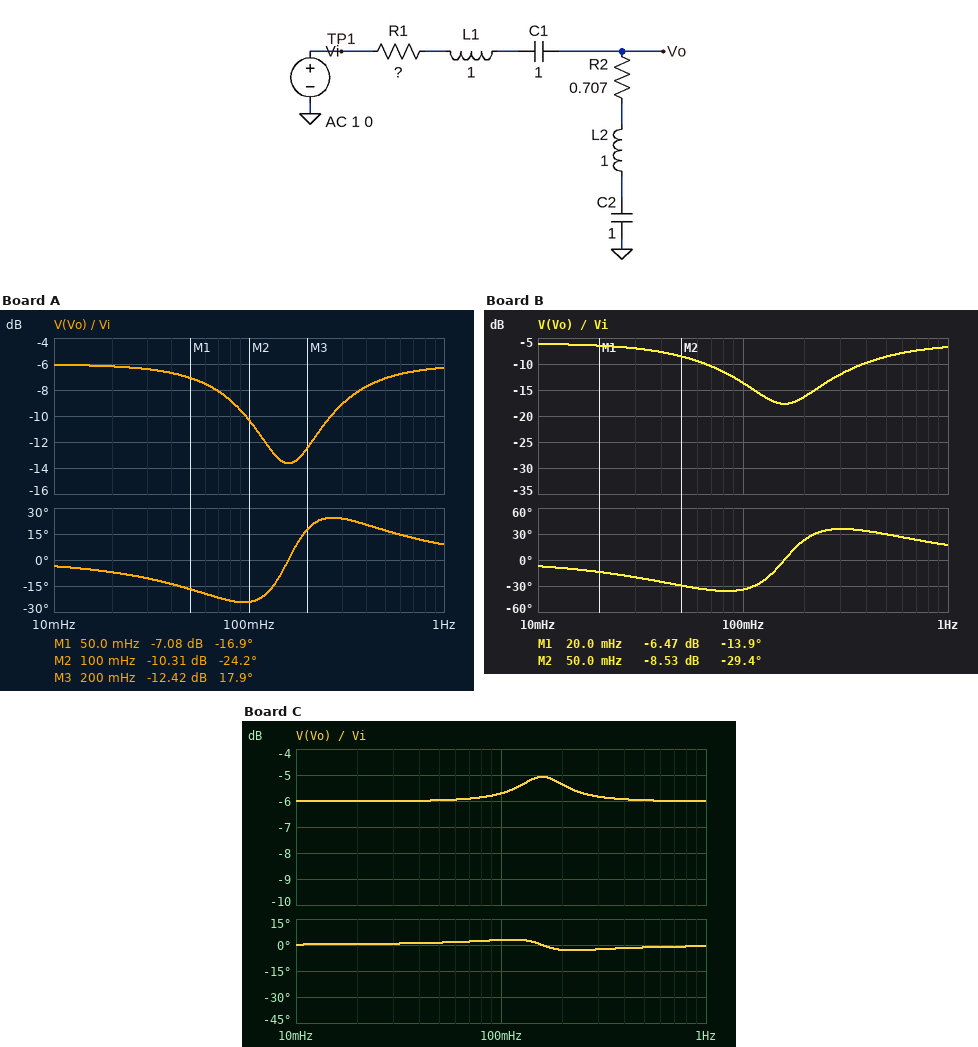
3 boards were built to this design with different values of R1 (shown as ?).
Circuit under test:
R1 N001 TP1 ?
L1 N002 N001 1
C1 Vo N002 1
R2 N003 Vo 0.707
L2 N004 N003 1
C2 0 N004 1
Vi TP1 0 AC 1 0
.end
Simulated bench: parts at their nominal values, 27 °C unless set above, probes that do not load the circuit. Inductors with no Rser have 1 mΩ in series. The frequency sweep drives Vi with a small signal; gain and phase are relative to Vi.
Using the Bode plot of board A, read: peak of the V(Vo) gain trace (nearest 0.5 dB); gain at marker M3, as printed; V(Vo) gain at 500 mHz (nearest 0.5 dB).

-6.0 dB
-12.42 dB
-7.0 dB
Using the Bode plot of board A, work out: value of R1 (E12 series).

2.7 Ω
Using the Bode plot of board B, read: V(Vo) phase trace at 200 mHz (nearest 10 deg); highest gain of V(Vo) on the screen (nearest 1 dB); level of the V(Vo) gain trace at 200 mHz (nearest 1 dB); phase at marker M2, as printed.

20 deg
-6 dB
-16 dB
-29.4 deg
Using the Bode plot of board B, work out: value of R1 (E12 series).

4.7 Ω
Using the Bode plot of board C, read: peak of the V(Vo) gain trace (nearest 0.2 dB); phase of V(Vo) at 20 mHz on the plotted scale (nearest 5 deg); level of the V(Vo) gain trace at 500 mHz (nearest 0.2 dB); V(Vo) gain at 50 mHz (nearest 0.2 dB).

-5.0 dB
0 deg
-6.0 dB
-6.0 dB
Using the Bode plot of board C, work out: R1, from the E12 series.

0.56 Ω
